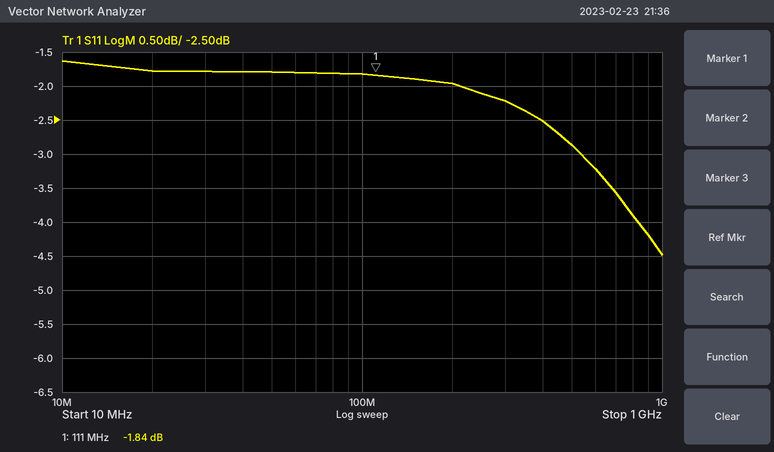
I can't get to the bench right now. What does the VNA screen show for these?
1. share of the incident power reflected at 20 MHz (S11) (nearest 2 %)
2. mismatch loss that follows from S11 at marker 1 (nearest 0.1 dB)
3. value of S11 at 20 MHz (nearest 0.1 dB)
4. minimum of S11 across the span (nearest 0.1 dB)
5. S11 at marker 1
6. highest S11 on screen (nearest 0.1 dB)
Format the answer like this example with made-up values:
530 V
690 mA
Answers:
66 %
4.6 dB
-1.8 dB
-4.5 dB
-1.84 dB
-1.6 dB
